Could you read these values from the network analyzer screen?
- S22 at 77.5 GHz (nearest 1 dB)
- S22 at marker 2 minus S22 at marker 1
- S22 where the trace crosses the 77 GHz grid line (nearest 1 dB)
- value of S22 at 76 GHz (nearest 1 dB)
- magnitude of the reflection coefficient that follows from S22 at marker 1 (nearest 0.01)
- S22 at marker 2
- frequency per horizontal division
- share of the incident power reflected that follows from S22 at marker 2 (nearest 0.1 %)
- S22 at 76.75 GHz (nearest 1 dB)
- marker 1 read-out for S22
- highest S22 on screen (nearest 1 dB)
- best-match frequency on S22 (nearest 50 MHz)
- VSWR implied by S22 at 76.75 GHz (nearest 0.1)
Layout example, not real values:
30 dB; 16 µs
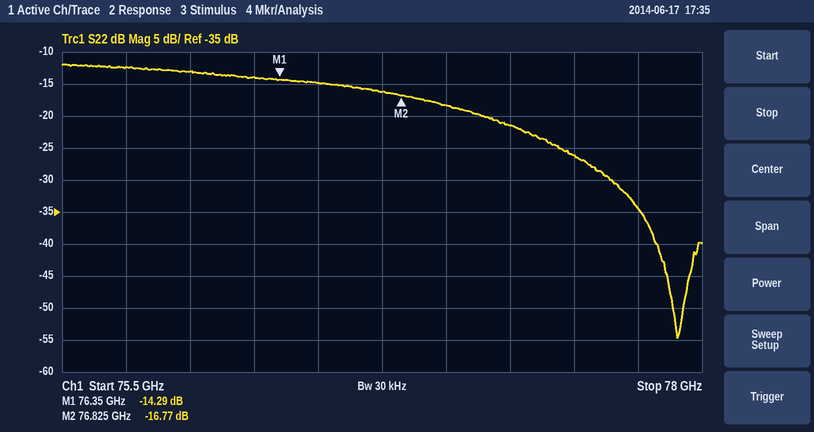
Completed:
-26 dB; -2.48 dB; -18 dB; -13 dB; 0.19; -16.77 dB; 250 MHz; 2.1 %; -16 dB; -14.29 dB; -12 dB; 77.90 GHz; 1.4
